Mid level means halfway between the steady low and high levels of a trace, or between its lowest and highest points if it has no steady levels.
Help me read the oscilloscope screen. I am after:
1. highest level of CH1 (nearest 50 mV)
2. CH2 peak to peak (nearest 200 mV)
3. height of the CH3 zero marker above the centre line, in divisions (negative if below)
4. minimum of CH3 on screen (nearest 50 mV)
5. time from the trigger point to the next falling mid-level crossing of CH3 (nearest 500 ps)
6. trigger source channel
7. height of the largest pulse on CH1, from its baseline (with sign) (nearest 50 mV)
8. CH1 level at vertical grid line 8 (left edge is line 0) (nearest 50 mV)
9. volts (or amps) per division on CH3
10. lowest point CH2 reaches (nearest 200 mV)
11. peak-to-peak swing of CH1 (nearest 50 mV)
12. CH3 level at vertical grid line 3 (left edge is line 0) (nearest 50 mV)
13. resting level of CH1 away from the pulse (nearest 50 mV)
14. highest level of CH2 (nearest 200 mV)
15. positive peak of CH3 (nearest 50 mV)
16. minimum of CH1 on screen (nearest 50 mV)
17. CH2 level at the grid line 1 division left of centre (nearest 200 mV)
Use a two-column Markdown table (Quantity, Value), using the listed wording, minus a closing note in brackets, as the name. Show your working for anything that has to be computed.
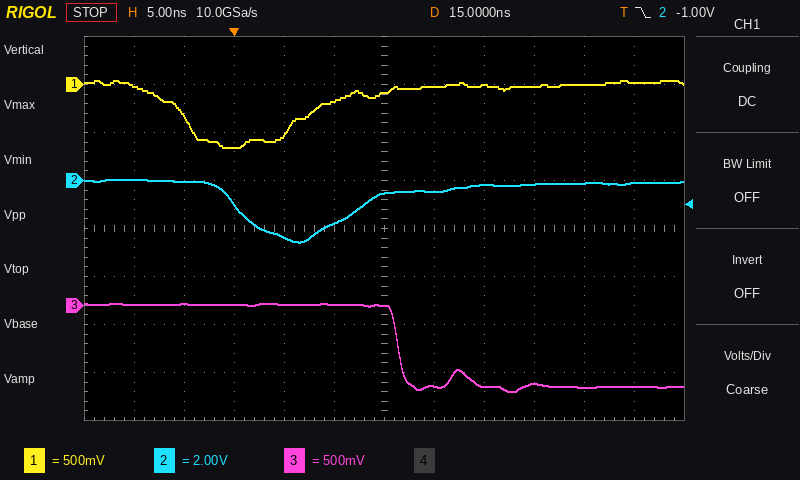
| Quantity | Value |
|---|---|
| highest level of CH1 | 50 mV |
| CH2 peak to peak | 0.0 V − (-2.6 V) = 2.6 V |
| height of the CH3 zero marker above the centre line, in divisions | -1.6 div |
| minimum of CH3 on screen | -900 mV |
| time from the trigger point to the next falling mid-level crossing of CH3 | 16.5 ns |
| trigger source channel | CH2 |
| height of the largest pulse on CH1, from its baseline (with sign) | -650 mV − (0 mV) = -650 mV |
| CH1 level at vertical grid line 8 (left edge is line 0) | 0 mV |
| volts (or amps) per division on CH3 | 500 mV |
| lowest point CH2 reaches | -2.6 V |
| peak-to-peak swing of CH1 | 50 mV − (-650 mV) = 700 mV |
| CH3 level at vertical grid line 3 (left edge is line 0) | 0 mV |
| resting level of CH1 away from the pulse | 0 mV |
| highest level of CH2 | 0.0 V |
| positive peak of CH3 | 0 mV |
| minimum of CH1 on screen | -650 mV |
| CH2 level at the grid line 1 division left of centre | -1.8 V |
